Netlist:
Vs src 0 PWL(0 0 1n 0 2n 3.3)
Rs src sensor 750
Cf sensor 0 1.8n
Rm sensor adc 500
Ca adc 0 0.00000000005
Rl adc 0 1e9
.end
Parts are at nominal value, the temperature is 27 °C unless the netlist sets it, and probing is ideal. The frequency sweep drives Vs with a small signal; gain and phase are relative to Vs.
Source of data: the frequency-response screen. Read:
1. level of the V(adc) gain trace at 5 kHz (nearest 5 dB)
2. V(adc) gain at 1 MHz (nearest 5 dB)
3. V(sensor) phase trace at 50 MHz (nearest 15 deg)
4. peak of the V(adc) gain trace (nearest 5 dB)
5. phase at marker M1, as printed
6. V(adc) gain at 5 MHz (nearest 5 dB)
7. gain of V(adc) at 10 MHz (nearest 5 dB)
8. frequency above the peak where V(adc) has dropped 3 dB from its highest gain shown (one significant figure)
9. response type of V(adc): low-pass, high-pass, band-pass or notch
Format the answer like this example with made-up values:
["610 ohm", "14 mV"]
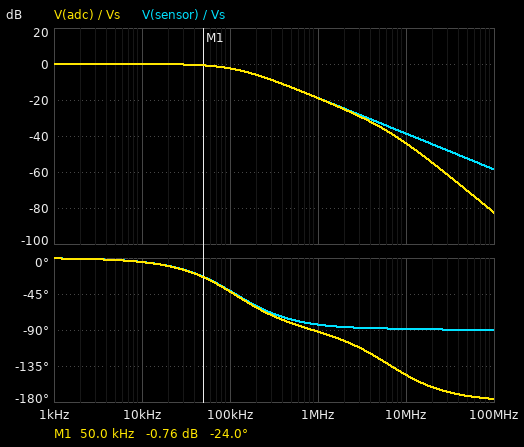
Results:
["0 dB", "-20 dB", "-90 deg", "0 dB", "-24.0 deg", "-35 dB", "-45 dB", "100 kHz", "low-pass"]
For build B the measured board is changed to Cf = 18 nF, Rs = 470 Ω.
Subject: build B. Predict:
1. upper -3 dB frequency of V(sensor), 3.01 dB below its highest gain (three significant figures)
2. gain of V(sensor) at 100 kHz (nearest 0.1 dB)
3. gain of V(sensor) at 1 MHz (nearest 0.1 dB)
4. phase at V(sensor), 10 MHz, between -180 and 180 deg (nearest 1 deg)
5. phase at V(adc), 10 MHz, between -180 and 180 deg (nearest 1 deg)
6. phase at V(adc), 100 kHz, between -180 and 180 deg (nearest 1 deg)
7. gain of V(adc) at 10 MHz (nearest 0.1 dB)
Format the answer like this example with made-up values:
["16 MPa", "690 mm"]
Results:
["18.8 kHz", "-14.7 dB", "-34.5 dB", "-90 deg", "-147 deg", "-80 deg", "-59.9 dB"]
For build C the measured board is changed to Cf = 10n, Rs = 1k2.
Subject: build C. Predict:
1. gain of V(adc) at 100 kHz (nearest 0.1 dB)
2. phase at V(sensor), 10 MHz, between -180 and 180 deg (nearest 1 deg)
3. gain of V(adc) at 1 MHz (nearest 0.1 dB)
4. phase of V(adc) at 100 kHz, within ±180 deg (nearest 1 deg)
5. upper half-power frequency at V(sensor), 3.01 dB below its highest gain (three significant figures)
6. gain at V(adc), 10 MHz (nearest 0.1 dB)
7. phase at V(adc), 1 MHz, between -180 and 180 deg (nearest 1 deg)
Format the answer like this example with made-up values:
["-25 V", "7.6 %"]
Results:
["-17.7 dB", "-90 deg", "-37.7 dB", "-83 deg", "13.2 kHz", "-63.0 dB", "-98 deg"]
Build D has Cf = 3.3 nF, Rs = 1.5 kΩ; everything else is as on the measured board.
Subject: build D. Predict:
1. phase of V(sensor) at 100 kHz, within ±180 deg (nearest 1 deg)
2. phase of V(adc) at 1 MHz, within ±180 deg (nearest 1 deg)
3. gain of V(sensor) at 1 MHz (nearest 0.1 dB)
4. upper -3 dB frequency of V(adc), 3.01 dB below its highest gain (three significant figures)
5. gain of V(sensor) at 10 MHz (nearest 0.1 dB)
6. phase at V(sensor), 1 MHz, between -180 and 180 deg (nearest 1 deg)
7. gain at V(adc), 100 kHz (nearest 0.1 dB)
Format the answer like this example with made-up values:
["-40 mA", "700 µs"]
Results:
["-72 deg", "-97 deg", "-30.0 dB", "31.7 kHz", "-49.9 dB", "-88 deg", "-10.4 dB"]
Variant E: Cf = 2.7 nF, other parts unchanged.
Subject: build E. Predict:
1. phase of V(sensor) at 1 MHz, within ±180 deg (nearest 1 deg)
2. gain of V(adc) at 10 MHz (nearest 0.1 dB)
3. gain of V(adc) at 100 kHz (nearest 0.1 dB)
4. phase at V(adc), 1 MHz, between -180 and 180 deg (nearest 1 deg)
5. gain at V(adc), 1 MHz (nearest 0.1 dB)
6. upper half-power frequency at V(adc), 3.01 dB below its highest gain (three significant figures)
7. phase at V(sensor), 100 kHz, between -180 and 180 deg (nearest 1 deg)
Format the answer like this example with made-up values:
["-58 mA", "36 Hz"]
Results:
["-85 deg", "-47.5 dB", "-4.3 dB", "-94 deg", "-22.4 dB", "77.1 kHz", "-52 deg"]
